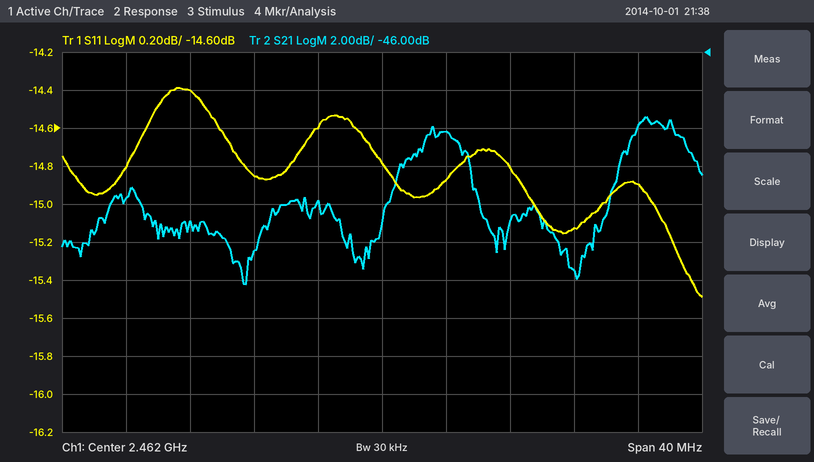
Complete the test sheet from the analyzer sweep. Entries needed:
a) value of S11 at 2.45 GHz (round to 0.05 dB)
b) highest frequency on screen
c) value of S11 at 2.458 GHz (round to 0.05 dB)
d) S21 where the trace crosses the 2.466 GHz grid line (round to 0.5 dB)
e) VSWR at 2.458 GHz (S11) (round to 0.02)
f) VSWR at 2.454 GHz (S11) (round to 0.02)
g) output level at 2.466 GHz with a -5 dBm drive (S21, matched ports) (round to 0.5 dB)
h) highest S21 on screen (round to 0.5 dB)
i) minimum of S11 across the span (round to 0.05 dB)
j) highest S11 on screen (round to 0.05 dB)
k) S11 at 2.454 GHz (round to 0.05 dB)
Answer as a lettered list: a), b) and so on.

a) -14.40 dB
b) 2.482 GHz
c) -14.60 dB
d) -50.0 dB
e) 1.46
f) 1.44
g) -55.0 dBm
h) -49.5 dB
i) -15.50 dB
j) -14.40 dB
k) -14.85 dB
